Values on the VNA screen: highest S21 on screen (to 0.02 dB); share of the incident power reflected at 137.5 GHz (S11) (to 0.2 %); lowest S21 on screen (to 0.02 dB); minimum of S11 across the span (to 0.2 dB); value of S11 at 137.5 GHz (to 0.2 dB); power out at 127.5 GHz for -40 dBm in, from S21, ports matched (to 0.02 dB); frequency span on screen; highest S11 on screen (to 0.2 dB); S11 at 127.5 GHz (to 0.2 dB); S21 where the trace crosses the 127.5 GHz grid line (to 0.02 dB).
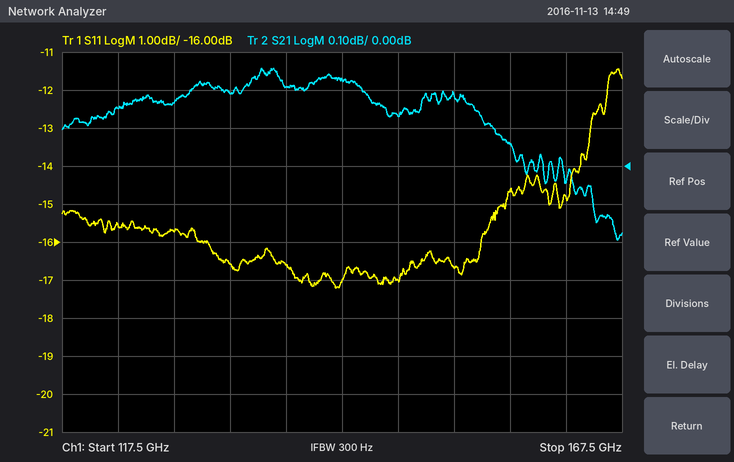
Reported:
0.26 dB
2.2 %
-0.20 dB
-17.2 dB
-16.6 dB
-39.84 dBm
50 GHz
-11.4 dB
-15.8 dB
0.16 dB
